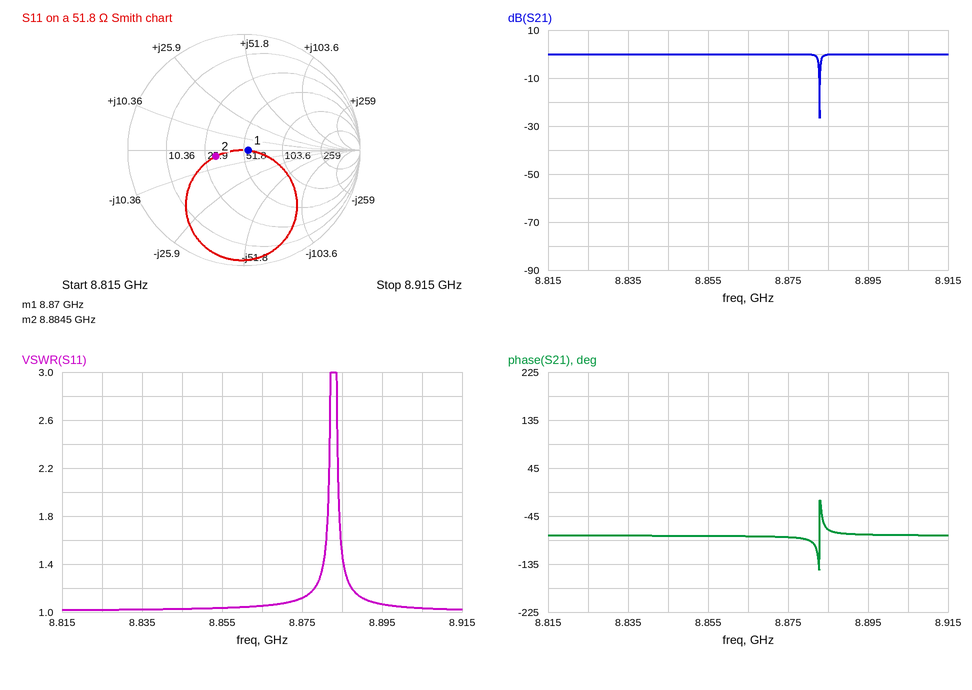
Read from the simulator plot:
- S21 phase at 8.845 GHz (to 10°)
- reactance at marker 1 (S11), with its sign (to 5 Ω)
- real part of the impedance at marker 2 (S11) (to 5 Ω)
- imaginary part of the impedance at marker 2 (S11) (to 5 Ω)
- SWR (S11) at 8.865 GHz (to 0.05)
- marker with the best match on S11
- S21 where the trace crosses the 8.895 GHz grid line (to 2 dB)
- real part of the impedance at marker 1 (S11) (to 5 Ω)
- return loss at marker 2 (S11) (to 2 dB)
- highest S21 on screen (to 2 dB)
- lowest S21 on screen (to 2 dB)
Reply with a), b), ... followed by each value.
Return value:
a) -80°
b) 0 Ω
c) 30 Ω
d) -5 Ω
e) 1.05
f) marker 1
g) 0 dB
h) 55 Ω
i) 12 dB
j) 0 dB
k) -26 dB
